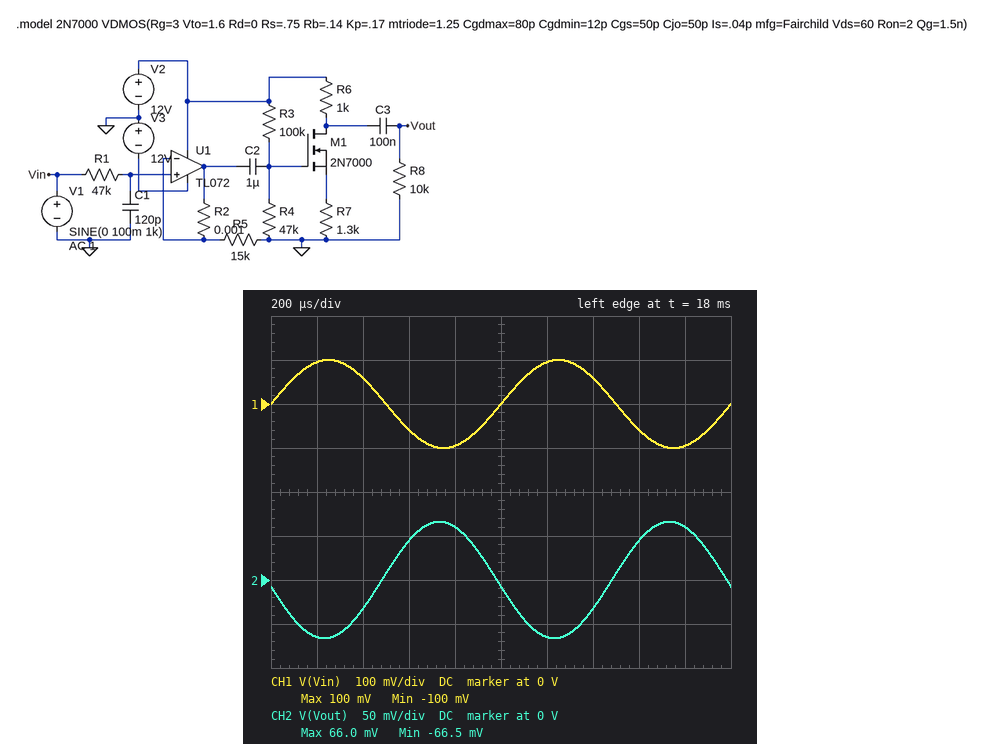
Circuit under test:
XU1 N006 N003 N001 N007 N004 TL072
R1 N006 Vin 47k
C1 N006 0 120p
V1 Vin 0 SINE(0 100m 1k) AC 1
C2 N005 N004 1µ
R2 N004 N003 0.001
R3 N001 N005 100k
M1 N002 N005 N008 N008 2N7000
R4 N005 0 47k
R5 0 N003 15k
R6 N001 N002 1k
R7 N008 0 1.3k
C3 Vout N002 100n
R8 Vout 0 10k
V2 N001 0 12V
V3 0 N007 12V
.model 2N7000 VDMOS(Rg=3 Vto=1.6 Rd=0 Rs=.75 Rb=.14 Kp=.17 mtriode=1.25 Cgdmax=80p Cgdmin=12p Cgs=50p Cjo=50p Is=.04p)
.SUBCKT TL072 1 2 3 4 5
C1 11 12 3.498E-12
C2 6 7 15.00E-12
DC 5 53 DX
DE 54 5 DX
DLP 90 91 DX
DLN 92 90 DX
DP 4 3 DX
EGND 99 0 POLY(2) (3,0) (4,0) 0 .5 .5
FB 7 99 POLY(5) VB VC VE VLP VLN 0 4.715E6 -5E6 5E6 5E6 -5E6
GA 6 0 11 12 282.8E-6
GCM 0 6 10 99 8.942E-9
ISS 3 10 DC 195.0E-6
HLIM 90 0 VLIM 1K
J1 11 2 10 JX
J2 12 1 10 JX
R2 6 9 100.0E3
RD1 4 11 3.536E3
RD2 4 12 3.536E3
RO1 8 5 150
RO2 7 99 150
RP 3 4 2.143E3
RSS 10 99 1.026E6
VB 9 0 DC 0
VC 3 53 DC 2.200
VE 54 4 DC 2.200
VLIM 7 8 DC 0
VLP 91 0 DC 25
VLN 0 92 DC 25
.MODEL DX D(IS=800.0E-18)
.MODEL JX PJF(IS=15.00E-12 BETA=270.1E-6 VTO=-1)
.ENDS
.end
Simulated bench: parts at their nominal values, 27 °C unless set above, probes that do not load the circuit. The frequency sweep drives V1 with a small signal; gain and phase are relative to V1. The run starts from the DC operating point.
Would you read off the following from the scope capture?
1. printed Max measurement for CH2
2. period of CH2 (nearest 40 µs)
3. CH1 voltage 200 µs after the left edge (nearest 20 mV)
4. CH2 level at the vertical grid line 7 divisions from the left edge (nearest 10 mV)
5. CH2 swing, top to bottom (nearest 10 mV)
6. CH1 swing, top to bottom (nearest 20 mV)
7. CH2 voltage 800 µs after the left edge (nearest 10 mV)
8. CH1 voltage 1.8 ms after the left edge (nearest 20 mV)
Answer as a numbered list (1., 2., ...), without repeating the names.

1. 66.0 mV
2. 1.00 ms
3. 100 mV
4. -30 mV
5. 130 mV
6. 200 mV
7. 60 mV
8. -100 mV
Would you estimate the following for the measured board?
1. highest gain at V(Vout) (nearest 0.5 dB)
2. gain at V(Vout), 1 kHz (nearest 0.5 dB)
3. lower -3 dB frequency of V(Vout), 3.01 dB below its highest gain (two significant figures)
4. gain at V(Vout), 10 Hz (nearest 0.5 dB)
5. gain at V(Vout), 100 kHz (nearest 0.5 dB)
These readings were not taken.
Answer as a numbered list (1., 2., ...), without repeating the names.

1. -3.5 dB
2. -3.5 dB
3. 140 Hz
4. -27.5 dB
5. -15.0 dB
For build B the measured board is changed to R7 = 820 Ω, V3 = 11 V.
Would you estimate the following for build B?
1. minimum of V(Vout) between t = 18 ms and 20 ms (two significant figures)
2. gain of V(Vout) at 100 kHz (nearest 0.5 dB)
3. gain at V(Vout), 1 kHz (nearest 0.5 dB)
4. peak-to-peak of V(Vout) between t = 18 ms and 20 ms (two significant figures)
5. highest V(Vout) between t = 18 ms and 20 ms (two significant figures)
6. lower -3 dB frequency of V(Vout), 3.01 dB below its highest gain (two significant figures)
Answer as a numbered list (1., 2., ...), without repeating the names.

1. -100 mV
2. -11.0 dB
3. 0.5 dB
4. 210 mV
5. 100 mV
6. 140 Hz
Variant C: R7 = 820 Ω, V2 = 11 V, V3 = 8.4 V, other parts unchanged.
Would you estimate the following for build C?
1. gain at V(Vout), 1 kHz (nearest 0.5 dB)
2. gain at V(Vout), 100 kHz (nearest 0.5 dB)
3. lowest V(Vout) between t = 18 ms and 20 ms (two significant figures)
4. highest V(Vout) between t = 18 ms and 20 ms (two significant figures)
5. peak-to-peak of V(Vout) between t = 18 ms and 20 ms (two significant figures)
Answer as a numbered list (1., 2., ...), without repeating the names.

1. 0.5 dB
2. -11.0 dB
3. -100 mV
4. 100 mV
5. 210 mV
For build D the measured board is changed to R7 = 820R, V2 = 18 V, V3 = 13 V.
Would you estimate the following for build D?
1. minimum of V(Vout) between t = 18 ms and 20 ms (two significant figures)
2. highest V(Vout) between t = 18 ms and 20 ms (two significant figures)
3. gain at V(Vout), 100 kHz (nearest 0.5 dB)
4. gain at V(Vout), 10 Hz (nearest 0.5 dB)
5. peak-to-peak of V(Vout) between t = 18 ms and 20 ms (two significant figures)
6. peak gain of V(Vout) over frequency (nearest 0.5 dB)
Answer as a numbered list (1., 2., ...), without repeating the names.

1. -110 mV
2. 110 mV
3. -10.5 dB
4. -23.5 dB
5. 210 mV
6. 0.5 dB
